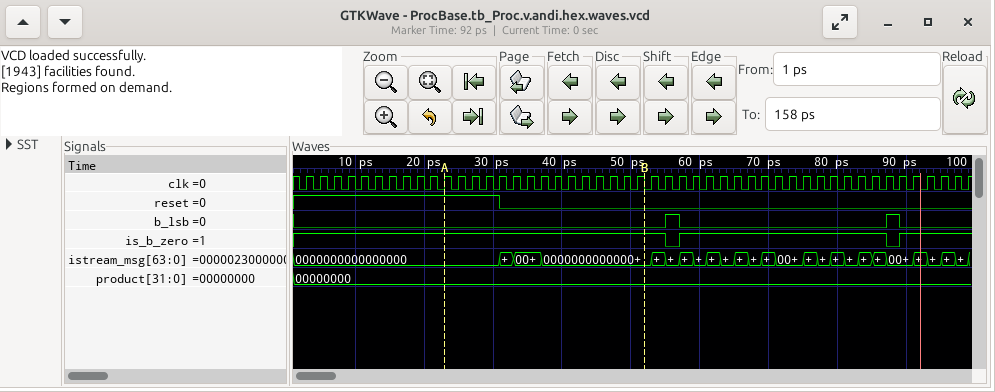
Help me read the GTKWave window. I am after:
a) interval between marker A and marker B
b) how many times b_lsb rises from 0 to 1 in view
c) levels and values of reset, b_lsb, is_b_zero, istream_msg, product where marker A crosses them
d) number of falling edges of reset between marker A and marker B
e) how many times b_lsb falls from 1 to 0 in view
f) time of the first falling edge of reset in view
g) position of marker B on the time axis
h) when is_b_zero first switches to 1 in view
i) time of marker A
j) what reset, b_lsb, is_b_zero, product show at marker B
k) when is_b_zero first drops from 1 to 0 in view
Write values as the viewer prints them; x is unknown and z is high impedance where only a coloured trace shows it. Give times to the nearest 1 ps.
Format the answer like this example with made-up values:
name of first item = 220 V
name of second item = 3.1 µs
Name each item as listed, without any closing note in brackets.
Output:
interval between marker A and marker B = 29 ps
how many times b_lsb rises from 0 to 1 in view = 2
levels and values of reset, b_lsb, is_b_zero, istream_msg, product where marker A crosses them = reset=1, b_lsb=0, is_b_zero=1, istream_msg=0000000000000000, product=00000000
number of falling edges of reset between marker A and marker B = 1
how many times b_lsb falls from 1 to 0 in view = 2
time of the first falling edge of reset in view = 31 ps
position of marker B on the time axis = 52 ps
when is_b_zero first switches to 1 in view = 57 ps
time of marker A = 23 ps
what reset, b_lsb, is_b_zero, product show at marker B = reset=0, b_lsb=0, is_b_zero=1, product=00000000
when is_b_zero first drops from 1 to 0 in view = 55 ps
